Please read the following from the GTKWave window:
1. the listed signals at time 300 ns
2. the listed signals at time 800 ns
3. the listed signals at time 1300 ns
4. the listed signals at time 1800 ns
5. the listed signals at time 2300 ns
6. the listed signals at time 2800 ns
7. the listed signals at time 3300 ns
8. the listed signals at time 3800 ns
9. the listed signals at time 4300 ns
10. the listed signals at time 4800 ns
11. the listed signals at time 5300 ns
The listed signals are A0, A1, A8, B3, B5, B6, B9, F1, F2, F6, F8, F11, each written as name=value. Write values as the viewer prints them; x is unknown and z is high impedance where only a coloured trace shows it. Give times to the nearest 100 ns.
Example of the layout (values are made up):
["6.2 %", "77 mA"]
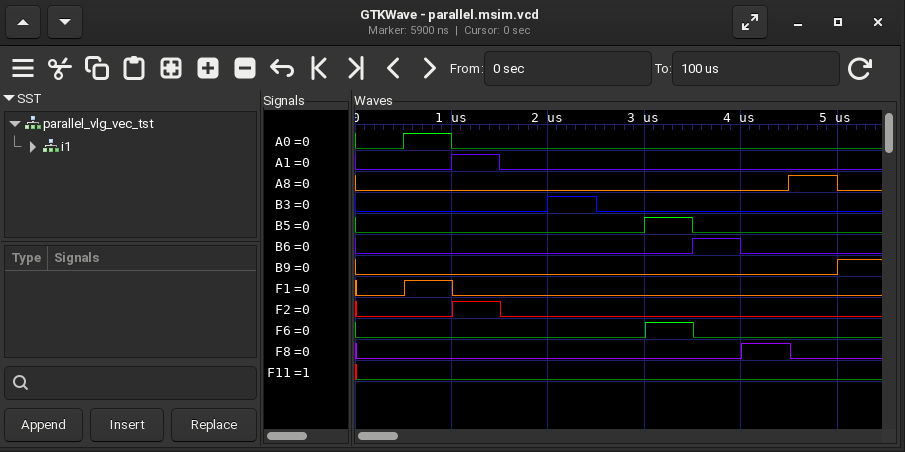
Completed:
["A0=0, A1=0, A8=0, B3=0, B5=0, B6=0, B9=0, F1=0, F2=0, F6=0, F8=0, F11=0", "A0=1, A1=0, A8=0, B3=0, B5=0, B6=0, B9=0, F1=1, F2=0, F6=0, F8=0, F11=0", "A0=0, A1=1, A8=0, B3=0, B5=0, B6=0, B9=0, F1=0, F2=1, F6=0, F8=0, F11=0", "A0=0, A1=0, A8=0, B3=0, B5=0, B6=0, B9=0, F1=0, F2=0, F6=0, F8=0, F11=0", "A0=0, A1=0, A8=0, B3=1, B5=0, B6=0, B9=0, F1=0, F2=0, F6=0, F8=0, F11=0", "A0=0, A1=0, A8=0, B3=0, B5=0, B6=0, B9=0, F1=0, F2=0, F6=0, F8=0, F11=0", "A0=0, A1=0, A8=0, B3=0, B5=1, B6=0, B9=0, F1=0, F2=0, F6=1, F8=0, F11=0", "A0=0, A1=0, A8=0, B3=0, B5=0, B6=1, B9=0, F1=0, F2=0, F6=0, F8=0, F11=0", "A0=0, A1=0, A8=0, B3=0, B5=0, B6=0, B9=0, F1=0, F2=0, F6=0, F8=1, F11=0", "A0=0, A1=0, A8=1, B3=0, B5=0, B6=0, B9=0, F1=0, F2=0, F6=0, F8=0, F11=0", "A0=0, A1=0, A8=0, B3=0, B5=0, B6=0, B9=1, F1=0, F2=0, F6=0, F8=0, F11=0"]
